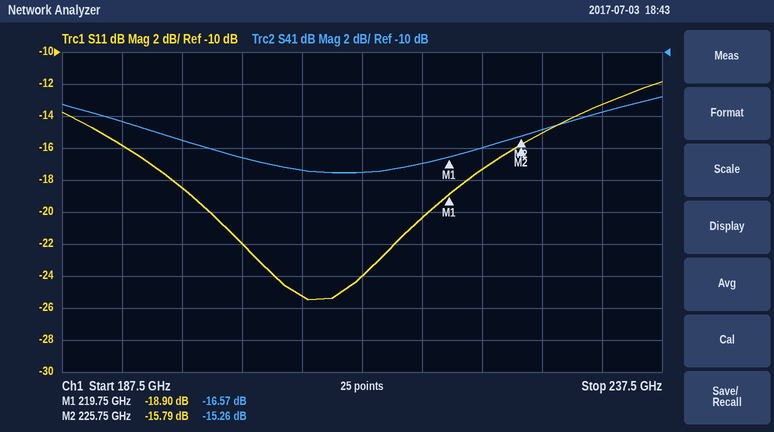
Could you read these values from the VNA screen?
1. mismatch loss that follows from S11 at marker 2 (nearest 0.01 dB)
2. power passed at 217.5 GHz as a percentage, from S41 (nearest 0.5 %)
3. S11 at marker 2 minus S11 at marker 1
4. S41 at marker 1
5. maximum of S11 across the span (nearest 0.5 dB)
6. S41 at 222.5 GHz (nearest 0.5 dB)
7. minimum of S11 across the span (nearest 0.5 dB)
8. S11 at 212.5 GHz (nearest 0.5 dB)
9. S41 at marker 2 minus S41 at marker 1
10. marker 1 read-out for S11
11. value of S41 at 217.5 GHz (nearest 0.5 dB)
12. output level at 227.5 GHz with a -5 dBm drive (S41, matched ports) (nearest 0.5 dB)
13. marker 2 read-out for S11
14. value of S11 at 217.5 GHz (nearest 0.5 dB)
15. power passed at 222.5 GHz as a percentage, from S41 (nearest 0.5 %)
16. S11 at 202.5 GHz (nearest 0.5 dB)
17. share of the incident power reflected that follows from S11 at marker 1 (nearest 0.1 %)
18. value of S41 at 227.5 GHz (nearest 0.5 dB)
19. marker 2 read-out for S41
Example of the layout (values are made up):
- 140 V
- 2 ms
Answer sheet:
- 0.12 dB
- 2.0 %
- 3.11 dB
- -16.57 dB
- -12.0 dB
- -16.0 dB
- -25.5 dB
- -24.0 dB
- 1.31 dB
- -18.90 dB
- -17.0 dB
- -20.0 dBm
- -15.79 dB
- -20.5 dB
- 2.5 %
- -22.0 dB
- 1.3 %
- -15.0 dB
- -15.26 dB
